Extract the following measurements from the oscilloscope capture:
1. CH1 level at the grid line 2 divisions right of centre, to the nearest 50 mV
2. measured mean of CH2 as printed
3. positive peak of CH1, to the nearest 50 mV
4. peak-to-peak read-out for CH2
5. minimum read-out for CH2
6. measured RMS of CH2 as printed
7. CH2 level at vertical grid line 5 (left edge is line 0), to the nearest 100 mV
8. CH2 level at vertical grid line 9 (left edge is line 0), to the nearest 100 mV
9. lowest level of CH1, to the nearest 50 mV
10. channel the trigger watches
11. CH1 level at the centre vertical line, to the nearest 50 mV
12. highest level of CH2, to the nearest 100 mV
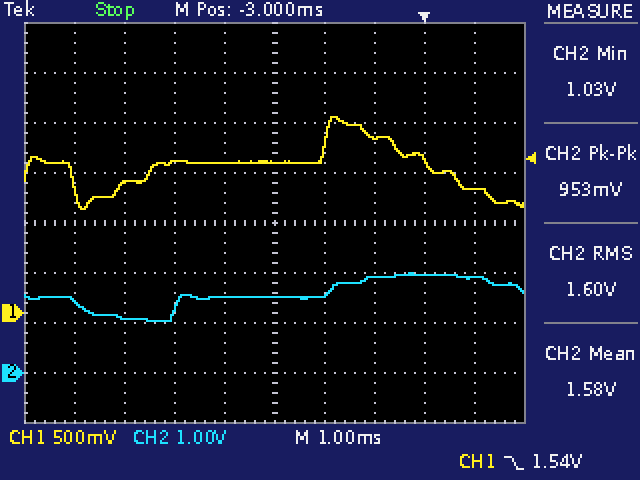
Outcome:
1.75 V
1.58 V
1.95 V
953 mV
1.03 V
1.60 V
1.5 V
1.9 V
1.05 V
CH1
1.50 V
2.0 V
